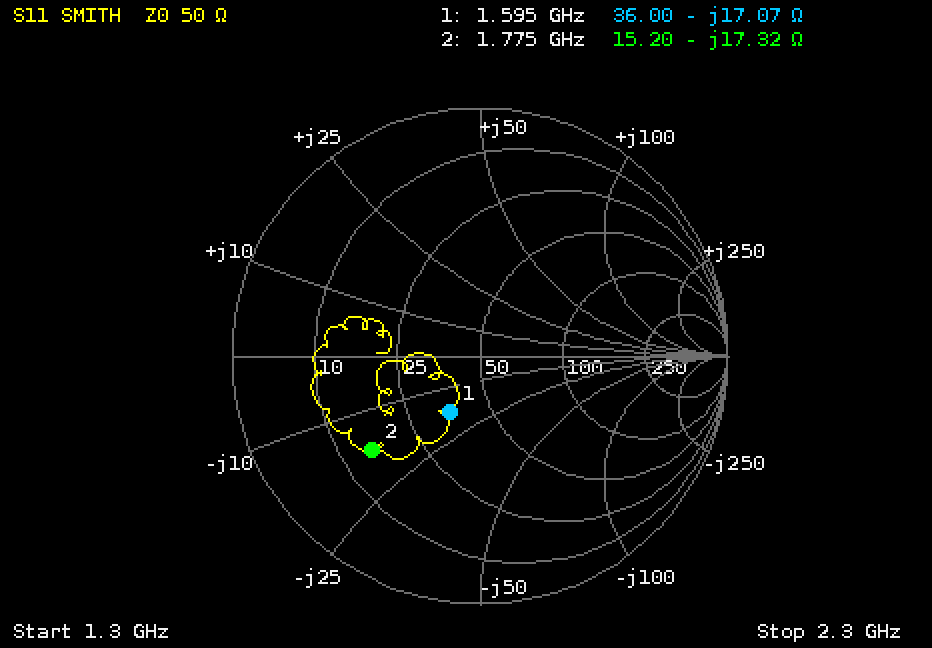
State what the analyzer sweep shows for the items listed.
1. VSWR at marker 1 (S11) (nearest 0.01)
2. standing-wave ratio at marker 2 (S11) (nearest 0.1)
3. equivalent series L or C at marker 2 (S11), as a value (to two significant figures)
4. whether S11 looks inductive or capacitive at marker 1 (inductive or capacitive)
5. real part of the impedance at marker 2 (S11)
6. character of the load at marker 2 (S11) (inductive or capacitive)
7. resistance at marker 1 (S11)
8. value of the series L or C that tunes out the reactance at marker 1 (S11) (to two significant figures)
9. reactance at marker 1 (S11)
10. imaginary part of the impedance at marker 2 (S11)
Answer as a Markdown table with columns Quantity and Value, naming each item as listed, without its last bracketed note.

| Quantity | Value |
|---|---|
| VSWR at marker 1 (S11) | 1.67 |
| standing-wave ratio at marker 2 (S11) | 3.7 |
| equivalent series L or C at marker 2 (S11), as a value | 5.2 pF |
| whether S11 looks inductive or capacitive at marker 1 | capacitive |
| real part of the impedance at marker 2 | 15.20 Ω |
| character of the load at marker 2 (S11) | capacitive |
| resistance at marker 1 | 36.00 Ω |
| value of the series L or C that tunes out the reactance at marker 1 (S11) | 1.7 nH |
| reactance at marker 1 | -17.07 Ω |
| imaginary part of the impedance at marker 2 | -17.32 Ω |
